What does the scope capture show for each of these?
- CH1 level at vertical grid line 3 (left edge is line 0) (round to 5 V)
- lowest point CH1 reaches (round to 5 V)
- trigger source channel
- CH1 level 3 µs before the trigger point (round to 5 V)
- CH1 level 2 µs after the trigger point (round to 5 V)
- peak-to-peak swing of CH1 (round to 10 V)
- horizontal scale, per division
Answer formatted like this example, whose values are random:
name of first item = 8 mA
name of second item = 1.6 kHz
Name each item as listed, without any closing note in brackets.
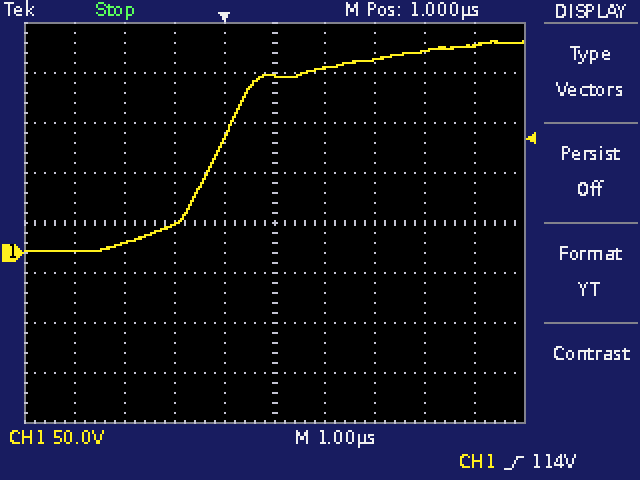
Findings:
CH1 level at vertical grid line 3 (left edge is line 0) = 30 V
lowest point CH1 reaches = 0 V
trigger source channel = CH1
CH1 level 3 µs before the trigger point = 0 V
CH1 level 2 µs after the trigger point = 185 V
peak-to-peak swing of CH1 = 210 V
horizontal scale, per division = 1 µs
